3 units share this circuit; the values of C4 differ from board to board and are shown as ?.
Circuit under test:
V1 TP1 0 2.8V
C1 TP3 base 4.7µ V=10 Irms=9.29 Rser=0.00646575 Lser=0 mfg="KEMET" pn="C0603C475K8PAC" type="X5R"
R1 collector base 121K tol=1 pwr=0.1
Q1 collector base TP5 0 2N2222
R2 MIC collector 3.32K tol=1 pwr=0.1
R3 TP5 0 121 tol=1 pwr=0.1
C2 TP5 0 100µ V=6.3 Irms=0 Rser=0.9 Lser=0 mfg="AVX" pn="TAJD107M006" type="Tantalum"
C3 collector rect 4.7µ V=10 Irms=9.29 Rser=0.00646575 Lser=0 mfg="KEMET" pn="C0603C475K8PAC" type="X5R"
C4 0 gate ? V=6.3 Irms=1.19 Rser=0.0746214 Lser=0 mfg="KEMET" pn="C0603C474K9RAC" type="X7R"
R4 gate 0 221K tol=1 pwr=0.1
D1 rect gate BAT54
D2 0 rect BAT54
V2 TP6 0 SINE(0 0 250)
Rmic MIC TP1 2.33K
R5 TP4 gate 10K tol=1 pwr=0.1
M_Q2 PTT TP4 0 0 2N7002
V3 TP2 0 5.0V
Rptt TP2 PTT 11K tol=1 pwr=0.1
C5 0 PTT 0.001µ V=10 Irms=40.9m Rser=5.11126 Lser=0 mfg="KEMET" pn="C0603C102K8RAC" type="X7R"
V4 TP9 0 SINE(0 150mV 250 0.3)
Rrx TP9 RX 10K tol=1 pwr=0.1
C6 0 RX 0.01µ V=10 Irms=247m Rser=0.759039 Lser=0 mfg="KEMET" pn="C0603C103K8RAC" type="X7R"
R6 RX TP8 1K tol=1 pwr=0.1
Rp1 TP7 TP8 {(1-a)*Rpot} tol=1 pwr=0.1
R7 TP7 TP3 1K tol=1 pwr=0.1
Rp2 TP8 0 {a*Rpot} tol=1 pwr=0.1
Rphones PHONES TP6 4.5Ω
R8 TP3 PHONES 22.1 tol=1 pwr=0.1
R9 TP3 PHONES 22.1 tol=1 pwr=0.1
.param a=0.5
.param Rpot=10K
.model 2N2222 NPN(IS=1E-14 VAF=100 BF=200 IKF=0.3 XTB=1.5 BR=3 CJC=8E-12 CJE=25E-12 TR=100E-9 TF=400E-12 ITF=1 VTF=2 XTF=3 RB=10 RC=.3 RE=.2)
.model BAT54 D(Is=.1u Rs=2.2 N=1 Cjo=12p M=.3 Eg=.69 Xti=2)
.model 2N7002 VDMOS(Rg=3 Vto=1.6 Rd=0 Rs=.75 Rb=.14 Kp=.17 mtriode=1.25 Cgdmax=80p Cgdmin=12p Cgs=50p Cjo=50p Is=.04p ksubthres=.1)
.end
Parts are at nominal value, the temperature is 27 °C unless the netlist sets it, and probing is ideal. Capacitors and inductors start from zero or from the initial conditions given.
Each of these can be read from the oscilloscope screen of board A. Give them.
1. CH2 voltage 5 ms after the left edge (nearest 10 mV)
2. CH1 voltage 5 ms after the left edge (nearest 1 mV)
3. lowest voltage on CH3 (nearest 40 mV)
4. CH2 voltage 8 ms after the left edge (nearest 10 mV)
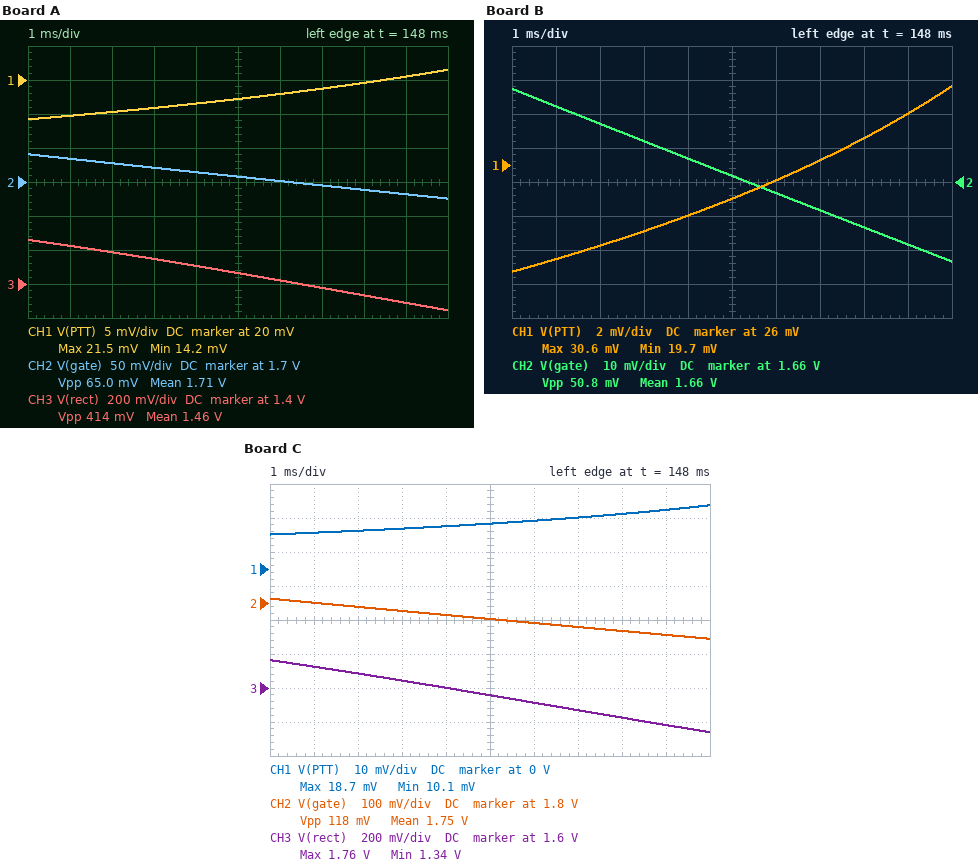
1.71 V
17 mV
1.24 V
1.69 V
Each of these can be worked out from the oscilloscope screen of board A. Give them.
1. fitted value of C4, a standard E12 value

1.2 µF
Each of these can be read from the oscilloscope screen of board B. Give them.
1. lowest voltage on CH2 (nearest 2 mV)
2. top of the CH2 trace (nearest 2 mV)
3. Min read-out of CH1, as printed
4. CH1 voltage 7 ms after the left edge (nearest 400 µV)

1.636 V
1.688 V
19.7 mV
26.4 mV
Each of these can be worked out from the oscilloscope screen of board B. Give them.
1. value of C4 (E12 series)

1.5 µF
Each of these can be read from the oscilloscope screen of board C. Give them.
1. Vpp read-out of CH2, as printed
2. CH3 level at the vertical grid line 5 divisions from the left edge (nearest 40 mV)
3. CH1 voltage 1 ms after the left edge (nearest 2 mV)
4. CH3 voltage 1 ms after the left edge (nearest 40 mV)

118 mV
1.56 V
10 mV
1.72 V
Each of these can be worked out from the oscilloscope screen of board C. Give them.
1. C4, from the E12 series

680 nF
